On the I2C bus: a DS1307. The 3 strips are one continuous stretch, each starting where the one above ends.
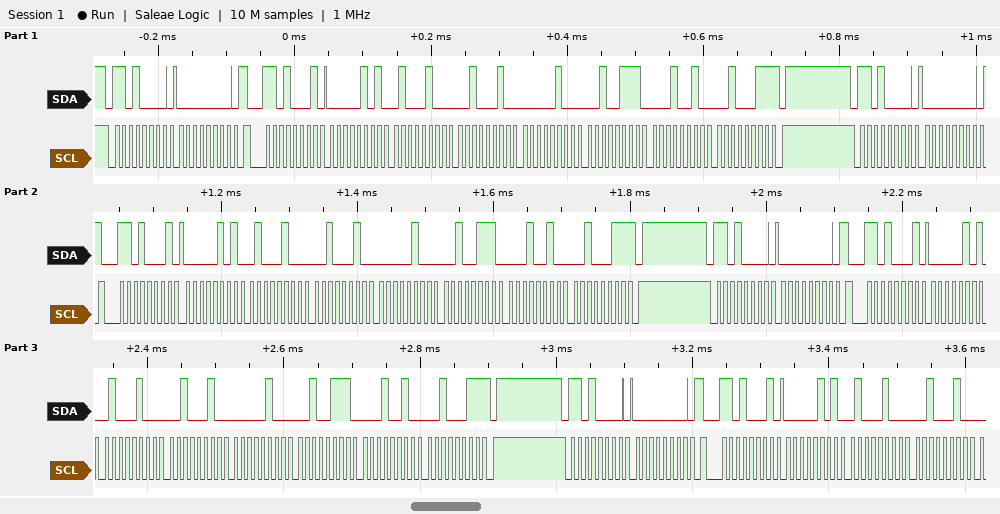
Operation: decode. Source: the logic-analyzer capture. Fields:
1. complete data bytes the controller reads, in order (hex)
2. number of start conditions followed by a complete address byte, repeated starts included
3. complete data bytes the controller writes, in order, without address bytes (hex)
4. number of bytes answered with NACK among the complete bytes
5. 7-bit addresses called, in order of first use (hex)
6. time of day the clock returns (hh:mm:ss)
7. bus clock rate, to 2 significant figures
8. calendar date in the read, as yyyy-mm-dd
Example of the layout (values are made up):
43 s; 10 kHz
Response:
05 44 22 04 27 12 23 05 44 22 04 27 12 23 05 44 22 04 27 12 23 05 44 22; 8; 00 00 00 00; 3; 0x68; 22:44:05; 100 kHz; 2023-12-27
